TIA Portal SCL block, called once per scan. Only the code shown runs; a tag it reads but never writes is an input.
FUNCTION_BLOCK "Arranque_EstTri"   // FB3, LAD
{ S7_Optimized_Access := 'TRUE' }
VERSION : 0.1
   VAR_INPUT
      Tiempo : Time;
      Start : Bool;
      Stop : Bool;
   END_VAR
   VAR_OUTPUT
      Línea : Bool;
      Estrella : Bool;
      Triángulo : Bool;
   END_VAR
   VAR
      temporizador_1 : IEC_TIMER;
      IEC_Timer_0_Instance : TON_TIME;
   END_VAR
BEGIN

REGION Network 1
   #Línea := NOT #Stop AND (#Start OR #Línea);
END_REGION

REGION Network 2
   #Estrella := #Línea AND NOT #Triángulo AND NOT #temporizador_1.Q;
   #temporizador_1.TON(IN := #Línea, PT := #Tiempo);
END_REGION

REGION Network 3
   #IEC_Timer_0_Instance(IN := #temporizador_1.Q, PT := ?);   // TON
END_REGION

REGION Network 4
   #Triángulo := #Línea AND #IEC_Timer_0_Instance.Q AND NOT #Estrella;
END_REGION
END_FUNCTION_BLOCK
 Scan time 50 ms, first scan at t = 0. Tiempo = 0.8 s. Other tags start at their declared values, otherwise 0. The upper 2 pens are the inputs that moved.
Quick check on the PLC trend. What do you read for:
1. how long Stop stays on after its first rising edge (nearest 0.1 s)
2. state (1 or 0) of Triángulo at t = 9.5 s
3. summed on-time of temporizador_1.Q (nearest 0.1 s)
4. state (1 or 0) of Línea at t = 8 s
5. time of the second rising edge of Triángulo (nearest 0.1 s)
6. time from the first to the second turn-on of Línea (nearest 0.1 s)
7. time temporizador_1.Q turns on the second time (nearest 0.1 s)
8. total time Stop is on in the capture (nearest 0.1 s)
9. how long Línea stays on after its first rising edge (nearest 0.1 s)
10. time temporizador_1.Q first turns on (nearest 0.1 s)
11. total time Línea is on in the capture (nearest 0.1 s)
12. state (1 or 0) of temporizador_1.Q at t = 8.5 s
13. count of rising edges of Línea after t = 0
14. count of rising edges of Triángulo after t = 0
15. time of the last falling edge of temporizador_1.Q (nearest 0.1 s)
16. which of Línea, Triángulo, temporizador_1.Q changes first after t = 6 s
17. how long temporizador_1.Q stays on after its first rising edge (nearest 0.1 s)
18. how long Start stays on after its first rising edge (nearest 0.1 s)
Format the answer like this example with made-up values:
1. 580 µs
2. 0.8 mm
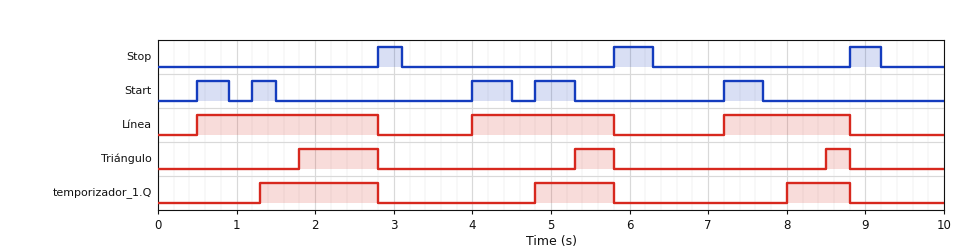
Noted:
1. 0.3 s
2. 0
3. 3.3 s
4. 1
5. 5.3 s
6. 3.5 s
7. 4.8 s
8. 1.2 s
9. 2.3 s
10. 1.3 s
11. 5.7 s
12. 1
13. 3
14. 3
15. 8.8 s
16. Línea
17. 1.5 s
18. 0.4 s
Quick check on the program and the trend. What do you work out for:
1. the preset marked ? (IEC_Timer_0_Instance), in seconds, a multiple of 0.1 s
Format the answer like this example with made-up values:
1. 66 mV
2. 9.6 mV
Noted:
1. 0.5 s
